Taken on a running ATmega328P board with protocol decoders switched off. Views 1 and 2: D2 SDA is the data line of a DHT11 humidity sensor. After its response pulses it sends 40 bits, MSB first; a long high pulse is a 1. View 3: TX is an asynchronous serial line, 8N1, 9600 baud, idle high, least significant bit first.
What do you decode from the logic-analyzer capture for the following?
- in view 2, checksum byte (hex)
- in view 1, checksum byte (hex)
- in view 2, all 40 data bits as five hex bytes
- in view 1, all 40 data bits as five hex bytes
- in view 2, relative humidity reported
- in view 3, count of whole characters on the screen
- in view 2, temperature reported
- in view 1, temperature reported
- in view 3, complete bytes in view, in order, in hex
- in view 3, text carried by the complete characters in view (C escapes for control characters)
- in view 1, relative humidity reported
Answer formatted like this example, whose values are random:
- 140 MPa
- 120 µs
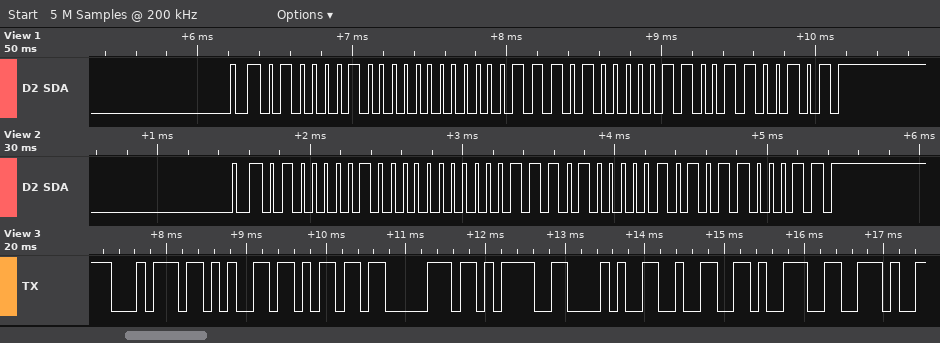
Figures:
- 0x63
- 0x65
- 41 00 1D 05 63
- 42 00 1D 06 65
- 65 %
- 9
- 29.5 °C
- 29.6 °C
- 74 65 6D 70 3D 28 32 39 2E
- "temp=(29."
- 66 %
